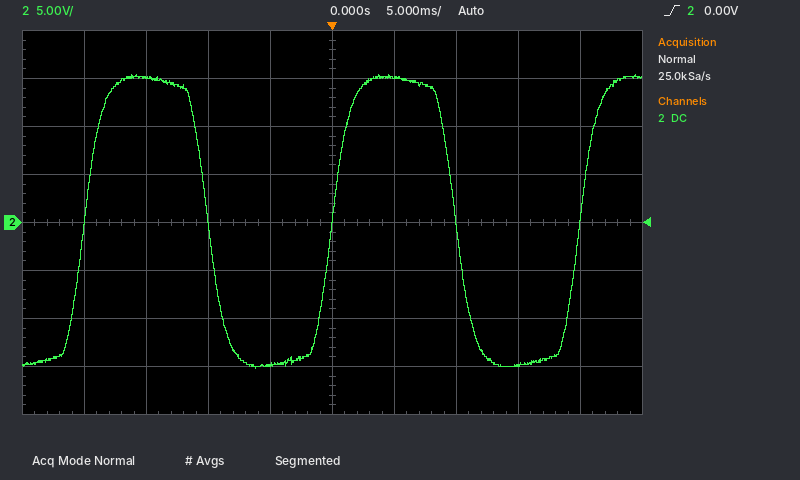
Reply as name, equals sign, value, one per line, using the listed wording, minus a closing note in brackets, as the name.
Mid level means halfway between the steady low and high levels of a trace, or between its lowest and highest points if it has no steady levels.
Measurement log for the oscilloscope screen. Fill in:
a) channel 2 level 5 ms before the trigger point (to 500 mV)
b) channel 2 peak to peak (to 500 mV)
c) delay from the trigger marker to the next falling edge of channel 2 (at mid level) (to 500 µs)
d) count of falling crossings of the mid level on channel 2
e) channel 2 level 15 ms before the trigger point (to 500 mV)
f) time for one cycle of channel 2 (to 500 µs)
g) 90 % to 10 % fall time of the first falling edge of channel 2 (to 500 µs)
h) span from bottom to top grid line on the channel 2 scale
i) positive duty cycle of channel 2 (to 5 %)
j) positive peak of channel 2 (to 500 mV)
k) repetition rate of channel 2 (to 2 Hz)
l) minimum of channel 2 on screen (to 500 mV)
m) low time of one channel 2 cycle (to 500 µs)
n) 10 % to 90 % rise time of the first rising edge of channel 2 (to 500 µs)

channel 2 level 5 ms before the trigger point = -15.0 V
channel 2 peak to peak = 30.5 V
delay from the trigger marker to the next falling edge of channel 2 (at mid level) = 10.0 ms
count of falling crossings of the mid level on channel 2 = 2
channel 2 level 15 ms before the trigger point = 15.0 V
time for one cycle of channel 2 = 20.0 ms
90 % to 10 % fall time of the first falling edge of channel 2 = 3.0 ms
span from bottom to top grid line on the channel 2 scale = 40 V
positive duty cycle of channel 2 = 50 %
positive peak of channel 2 = 15.5 V
repetition rate of channel 2 = 50 Hz
minimum of channel 2 on screen = -15.0 V
low time of one channel 2 cycle = 10.0 ms
10 % to 90 % rise time of the first rising edge of channel 2 = 3.0 ms
